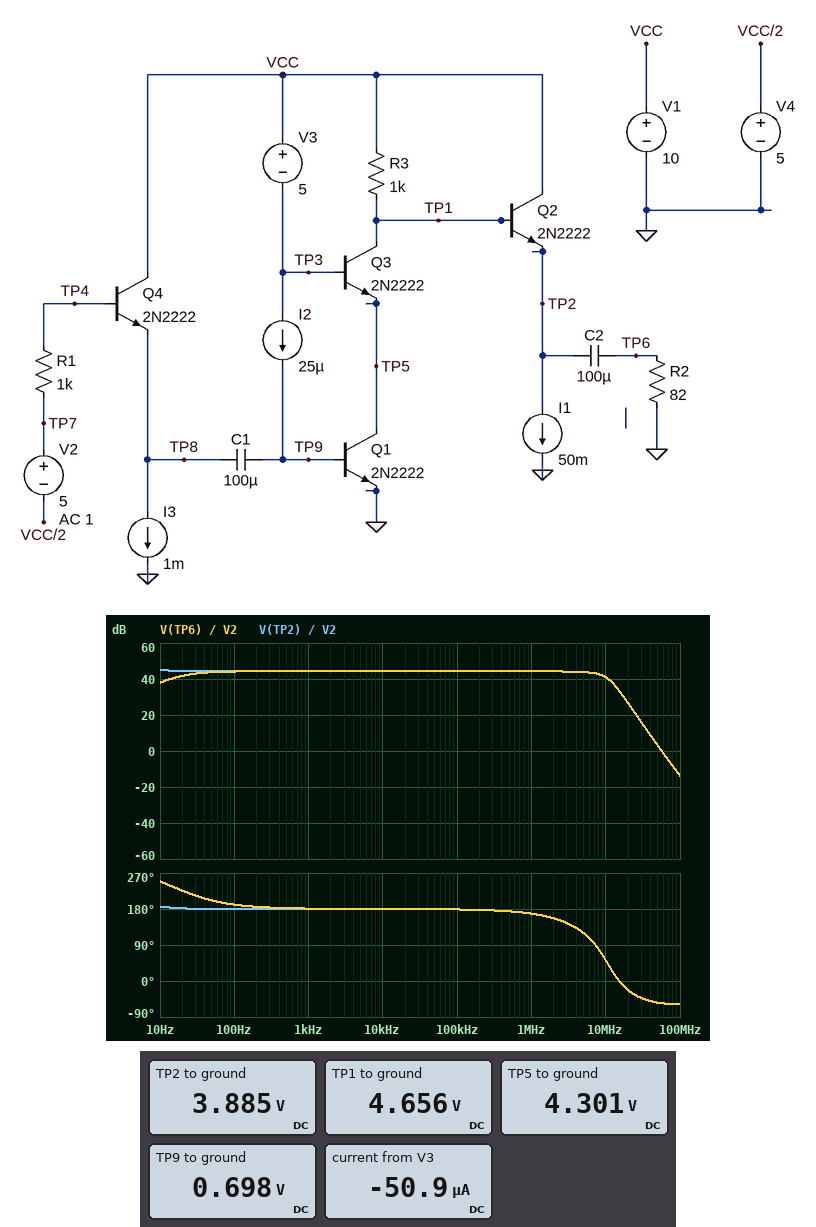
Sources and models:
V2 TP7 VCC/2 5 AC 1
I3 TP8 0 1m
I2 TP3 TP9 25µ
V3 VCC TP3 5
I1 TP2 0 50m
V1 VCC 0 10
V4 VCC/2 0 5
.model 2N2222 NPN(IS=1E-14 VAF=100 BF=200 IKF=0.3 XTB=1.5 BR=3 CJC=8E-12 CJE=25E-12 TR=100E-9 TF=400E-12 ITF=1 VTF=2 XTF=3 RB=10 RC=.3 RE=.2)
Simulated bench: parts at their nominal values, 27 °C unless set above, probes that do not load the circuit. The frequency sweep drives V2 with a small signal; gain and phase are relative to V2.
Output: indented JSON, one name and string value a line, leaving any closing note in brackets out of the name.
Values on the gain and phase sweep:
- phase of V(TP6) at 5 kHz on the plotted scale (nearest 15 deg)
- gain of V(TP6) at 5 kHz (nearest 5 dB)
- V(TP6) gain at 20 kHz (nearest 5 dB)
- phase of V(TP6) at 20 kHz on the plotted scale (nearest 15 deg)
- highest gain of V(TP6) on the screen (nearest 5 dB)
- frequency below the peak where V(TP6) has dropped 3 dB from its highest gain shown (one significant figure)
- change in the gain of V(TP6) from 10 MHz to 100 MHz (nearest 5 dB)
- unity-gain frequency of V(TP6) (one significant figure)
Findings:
{
  "phase of V(TP6) at 5 kHz on the plotted scale": "180 deg",
  "gain of V(TP6) at 5 kHz": "45 dB",
  "V(TP6) gain at 20 kHz": "45 dB",
  "phase of V(TP6) at 20 kHz on the plotted scale": "180 deg",
  "highest gain of V(TP6) on the screen": "45 dB",
  "frequency below the peak where V(TP6) has dropped 3 dB from its highest gain shown": "20 Hz",
  "change in the gain of V(TP6) from 10 MHz to 100 MHz": "-55 dB",
  "unity-gain frequency of V(TP6)": "60 MHz"
}
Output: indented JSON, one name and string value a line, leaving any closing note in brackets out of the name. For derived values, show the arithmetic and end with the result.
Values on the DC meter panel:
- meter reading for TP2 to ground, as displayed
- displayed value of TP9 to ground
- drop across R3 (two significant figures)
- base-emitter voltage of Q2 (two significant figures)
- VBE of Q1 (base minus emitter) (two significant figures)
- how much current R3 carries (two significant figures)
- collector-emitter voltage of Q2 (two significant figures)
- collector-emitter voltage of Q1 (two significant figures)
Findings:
{
  "meter reading for TP2 to ground, as displayed": "3.885 V",
  "displayed value of TP9 to ground": "0.698 V",
  "drop across R3": "10 V - 4.656 V = 5.3 V",
  "base-emitter voltage of Q2": "4.656 V - 3.885 V = 770 mV",
  "VBE of Q1 (base minus emitter)": "698 mV = 700 mV",
  "how much current R3 carries": "(10 V - 4.656 V) / 1 kΩ = 5.3 mA",
  "collector-emitter voltage of Q2": "10 V - 3.885 V = 6.1 V",
  "collector-emitter voltage of Q1": "4.301 V = 4.3 V"
}
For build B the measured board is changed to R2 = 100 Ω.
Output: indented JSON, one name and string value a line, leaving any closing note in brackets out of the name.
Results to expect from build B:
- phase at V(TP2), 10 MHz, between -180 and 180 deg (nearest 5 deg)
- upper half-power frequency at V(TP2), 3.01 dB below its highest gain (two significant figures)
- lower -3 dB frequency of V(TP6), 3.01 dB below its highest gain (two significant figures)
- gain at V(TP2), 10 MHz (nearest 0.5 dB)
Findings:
{
  "phase at V(TP2), 10 MHz, between -180 and 180 deg": "55 deg",
  "upper half-power frequency at V(TP2), 3.01 dB below its highest gain": "9.6 MHz",
  "lower -3 dB frequency of V(TP6), 3.01 dB below its highest gain": "15 Hz",
  "gain at V(TP2), 10 MHz": "41.5 dB"
}
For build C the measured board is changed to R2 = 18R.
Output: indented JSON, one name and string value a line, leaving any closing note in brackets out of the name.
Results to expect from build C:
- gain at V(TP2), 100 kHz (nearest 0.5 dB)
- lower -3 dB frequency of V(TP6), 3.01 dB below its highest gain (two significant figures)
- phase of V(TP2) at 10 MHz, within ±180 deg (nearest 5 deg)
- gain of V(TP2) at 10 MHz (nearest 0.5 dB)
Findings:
{
  "gain at V(TP2), 100 kHz": "42.0 dB",
  "lower -3 dB frequency of V(TP6), 3.01 dB below its highest gain": "64 Hz",
  "phase of V(TP2) at 10 MHz, within ±180 deg": "40 deg",
  "gain of V(TP2) at 10 MHz": "36.5 dB"
}
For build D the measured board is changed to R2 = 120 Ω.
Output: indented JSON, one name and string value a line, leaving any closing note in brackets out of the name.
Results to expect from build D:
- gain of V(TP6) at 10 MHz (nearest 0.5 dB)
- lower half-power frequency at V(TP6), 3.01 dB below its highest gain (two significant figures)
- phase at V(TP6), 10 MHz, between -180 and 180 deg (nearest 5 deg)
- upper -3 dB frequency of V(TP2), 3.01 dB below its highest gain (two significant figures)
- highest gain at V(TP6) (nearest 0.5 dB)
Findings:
{
  "gain of V(TP6) at 10 MHz": "41.5 dB",
  "lower half-power frequency at V(TP6), 3.01 dB below its highest gain": "13 Hz",
  "phase at V(TP6), 10 MHz, between -180 and 180 deg": "55 deg",
  "upper -3 dB frequency of V(TP2), 3.01 dB below its highest gain": "9.8 MHz",
  "highest gain at V(TP6)": "44.5 dB"
}
